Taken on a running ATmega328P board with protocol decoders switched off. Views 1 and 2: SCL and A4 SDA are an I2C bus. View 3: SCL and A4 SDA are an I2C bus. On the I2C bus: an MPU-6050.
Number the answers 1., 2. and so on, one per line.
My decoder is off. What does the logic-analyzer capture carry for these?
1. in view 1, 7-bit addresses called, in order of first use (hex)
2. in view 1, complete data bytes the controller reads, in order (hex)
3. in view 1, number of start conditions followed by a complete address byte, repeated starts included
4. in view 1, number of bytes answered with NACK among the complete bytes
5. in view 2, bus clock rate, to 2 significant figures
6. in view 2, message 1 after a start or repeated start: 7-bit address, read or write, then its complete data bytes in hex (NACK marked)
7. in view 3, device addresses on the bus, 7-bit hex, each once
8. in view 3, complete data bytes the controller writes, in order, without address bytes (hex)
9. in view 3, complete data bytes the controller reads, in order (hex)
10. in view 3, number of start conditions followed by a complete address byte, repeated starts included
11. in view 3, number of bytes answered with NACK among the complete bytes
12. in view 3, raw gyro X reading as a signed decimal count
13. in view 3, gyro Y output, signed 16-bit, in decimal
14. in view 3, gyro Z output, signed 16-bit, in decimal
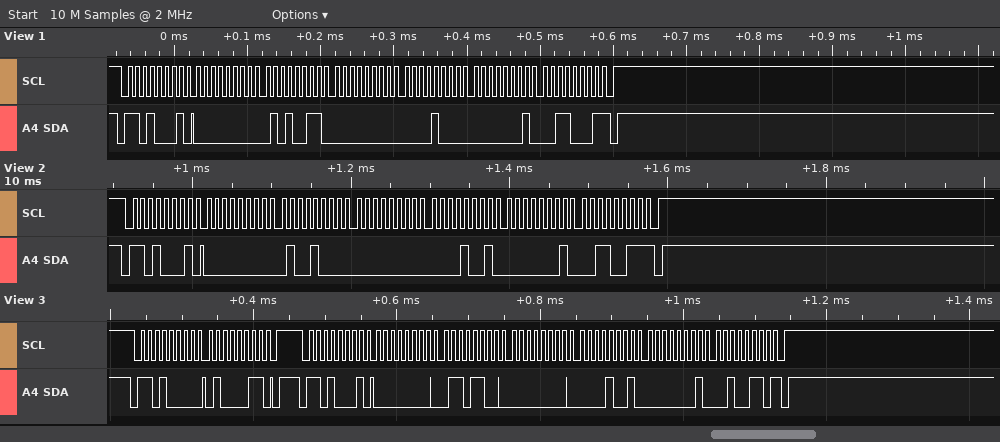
1. 0x68
2. 00 53 00 08 01 31
3. 1
4. 1
5. 100 kHz
6. 0x68 read: 00 48 00 09 01 33 NACK
7. 0x68
8. 43
9. 00 6C 00 09 01 26
10. 2
11. 1
12. 108
13. 9
14. 294
